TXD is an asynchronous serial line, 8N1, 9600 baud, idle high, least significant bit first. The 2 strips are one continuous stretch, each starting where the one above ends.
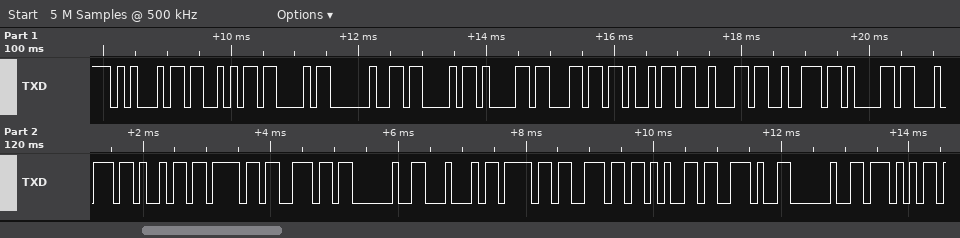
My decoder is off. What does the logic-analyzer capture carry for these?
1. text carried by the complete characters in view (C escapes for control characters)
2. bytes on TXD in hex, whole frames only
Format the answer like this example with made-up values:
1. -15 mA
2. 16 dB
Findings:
1. "ESC Calibration Done. W"
2. 45 53 43 20 43 61 6C 69 62 72 61 74 69 6F 6E 20 44 6F 6E 65 2E 20 57
